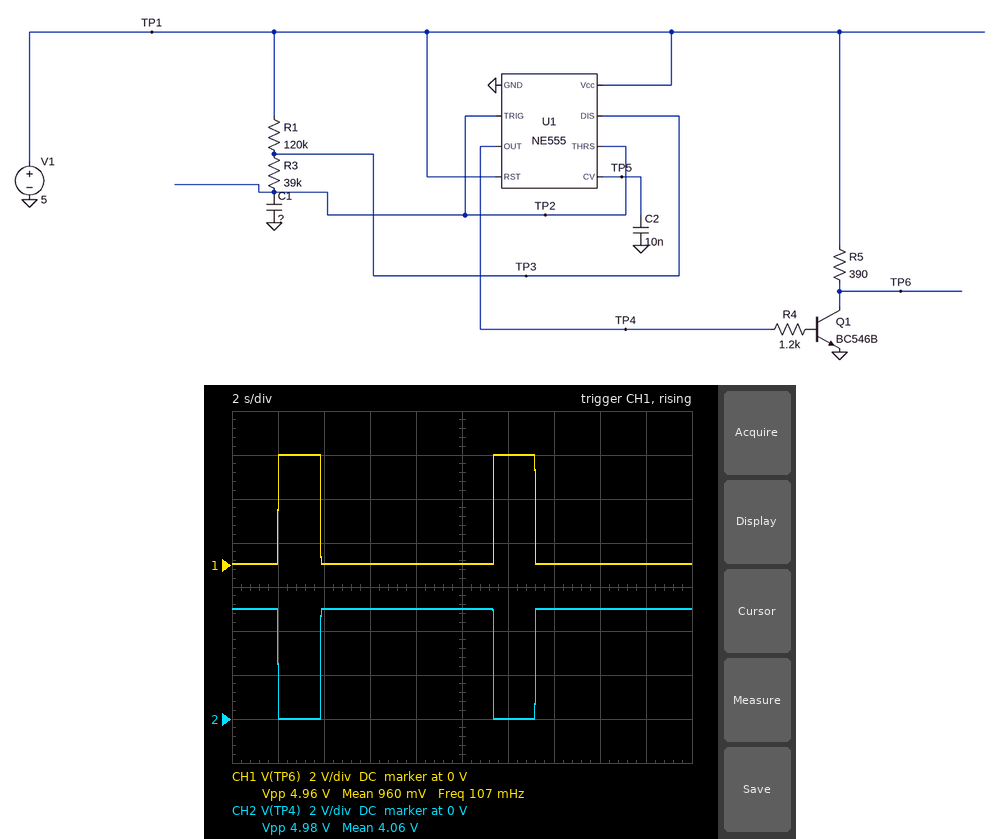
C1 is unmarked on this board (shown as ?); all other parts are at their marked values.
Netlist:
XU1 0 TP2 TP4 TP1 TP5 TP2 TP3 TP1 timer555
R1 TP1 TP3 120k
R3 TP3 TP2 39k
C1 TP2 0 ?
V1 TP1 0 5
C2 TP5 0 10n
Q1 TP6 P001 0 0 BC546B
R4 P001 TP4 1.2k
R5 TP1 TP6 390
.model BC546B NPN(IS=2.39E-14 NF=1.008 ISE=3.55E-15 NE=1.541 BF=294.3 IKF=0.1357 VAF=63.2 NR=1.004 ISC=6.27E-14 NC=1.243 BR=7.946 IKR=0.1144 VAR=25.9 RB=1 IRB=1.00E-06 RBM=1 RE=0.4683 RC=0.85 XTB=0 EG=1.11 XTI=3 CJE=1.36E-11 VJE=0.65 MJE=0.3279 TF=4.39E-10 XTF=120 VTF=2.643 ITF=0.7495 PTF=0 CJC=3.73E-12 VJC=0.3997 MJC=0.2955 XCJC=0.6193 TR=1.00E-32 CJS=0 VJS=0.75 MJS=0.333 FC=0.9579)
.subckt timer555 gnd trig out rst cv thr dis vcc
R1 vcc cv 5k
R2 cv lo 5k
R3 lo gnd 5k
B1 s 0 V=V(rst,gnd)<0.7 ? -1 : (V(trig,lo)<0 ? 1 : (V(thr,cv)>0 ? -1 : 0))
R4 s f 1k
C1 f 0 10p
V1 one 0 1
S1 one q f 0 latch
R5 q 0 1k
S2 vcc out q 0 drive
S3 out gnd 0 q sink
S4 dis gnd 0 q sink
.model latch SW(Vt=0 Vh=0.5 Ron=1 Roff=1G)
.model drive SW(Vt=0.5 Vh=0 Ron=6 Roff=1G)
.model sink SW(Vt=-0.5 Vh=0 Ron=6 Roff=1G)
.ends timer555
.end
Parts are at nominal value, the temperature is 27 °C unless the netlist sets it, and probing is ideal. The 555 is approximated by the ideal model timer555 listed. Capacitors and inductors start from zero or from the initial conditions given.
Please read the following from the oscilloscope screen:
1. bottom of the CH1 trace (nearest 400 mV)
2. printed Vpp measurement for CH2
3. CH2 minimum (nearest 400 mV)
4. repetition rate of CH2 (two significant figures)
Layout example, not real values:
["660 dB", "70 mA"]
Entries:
["0 V", "4.98 V", "0 V", "110 mHz"]
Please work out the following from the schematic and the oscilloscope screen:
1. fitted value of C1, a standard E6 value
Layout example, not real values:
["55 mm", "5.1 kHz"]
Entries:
["68 µF"]
